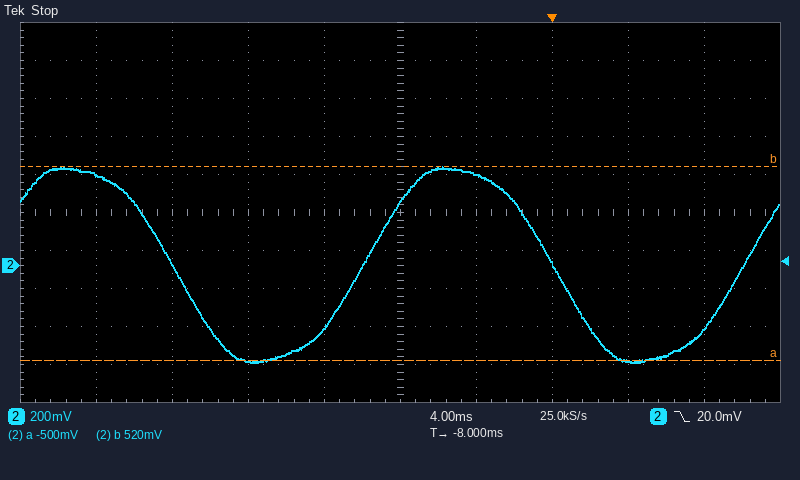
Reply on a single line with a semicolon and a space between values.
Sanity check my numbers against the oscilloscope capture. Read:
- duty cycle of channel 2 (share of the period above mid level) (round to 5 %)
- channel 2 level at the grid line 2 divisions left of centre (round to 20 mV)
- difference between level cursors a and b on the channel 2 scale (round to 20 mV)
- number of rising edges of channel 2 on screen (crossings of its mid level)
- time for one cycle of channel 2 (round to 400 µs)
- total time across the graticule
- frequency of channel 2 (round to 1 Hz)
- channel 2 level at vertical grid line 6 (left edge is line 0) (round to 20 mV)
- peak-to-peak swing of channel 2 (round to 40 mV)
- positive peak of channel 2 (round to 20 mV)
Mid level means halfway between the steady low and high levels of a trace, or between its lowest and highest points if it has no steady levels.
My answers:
50 %; -500 mV; 1.02 V; 2; 20.0 ms; 40 ms; 50 Hz; 480 mV; 1.04 V; 520 mV
